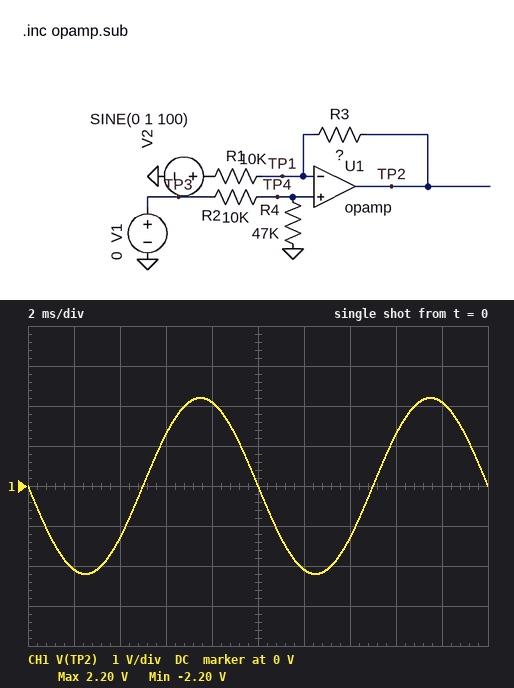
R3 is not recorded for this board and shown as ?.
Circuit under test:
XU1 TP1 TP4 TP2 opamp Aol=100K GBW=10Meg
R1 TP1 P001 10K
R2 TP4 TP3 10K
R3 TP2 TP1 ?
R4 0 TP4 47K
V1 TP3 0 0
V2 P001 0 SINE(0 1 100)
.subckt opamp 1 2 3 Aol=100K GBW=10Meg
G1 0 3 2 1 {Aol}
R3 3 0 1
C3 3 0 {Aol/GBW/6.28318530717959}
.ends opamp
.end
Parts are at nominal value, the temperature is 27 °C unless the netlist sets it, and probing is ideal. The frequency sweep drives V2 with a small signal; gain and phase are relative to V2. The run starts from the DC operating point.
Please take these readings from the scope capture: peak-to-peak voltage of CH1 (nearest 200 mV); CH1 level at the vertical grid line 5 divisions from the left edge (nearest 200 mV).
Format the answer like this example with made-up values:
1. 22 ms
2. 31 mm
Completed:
1. 4.4 V
2. 0 V
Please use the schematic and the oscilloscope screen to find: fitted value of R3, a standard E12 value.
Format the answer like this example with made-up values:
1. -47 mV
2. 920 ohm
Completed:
1. 22 kΩ
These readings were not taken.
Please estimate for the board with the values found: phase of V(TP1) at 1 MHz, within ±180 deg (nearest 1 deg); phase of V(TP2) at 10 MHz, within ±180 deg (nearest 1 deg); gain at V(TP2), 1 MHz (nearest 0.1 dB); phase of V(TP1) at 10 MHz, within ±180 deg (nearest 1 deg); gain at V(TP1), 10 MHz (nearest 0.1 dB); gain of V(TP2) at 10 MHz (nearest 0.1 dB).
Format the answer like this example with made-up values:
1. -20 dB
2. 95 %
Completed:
1. 72 deg
2. 107 deg
3. 6.4 dB
4. 17 deg
5. -3.7 dB
6. -3.7 dB
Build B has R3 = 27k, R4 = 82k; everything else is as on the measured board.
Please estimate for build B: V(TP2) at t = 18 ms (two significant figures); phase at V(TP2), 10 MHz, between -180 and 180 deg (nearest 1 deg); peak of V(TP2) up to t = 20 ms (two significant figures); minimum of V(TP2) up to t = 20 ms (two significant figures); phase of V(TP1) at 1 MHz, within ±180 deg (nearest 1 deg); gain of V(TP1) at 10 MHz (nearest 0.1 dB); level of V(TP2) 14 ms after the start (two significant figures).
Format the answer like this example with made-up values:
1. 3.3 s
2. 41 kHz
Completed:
1. 2.6 V
2. 105 deg
3. 2.7 V
4. -2.7 V
5. 70 deg
6. -3.0 dB
7. -1.6 V
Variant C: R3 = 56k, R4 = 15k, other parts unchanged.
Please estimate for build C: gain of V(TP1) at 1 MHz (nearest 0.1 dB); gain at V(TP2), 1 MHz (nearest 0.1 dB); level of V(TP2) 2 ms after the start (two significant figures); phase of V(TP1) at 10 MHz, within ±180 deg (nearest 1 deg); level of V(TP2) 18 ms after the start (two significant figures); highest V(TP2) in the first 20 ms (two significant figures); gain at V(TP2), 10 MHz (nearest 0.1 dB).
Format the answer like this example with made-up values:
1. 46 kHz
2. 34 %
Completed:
1. -6.6 dB
2. 13.4 dB
3. -5.3 V
4. 9 deg
5. 5.3 V
6. 5.6 V
7. -1.5 dB
